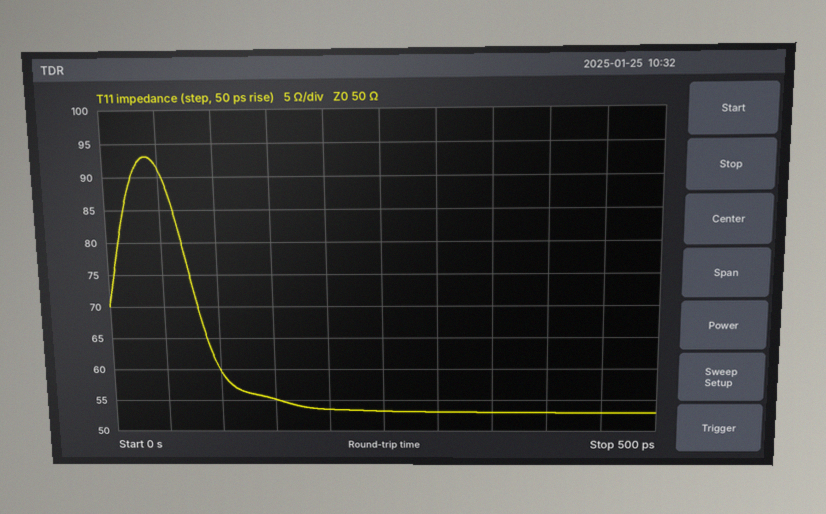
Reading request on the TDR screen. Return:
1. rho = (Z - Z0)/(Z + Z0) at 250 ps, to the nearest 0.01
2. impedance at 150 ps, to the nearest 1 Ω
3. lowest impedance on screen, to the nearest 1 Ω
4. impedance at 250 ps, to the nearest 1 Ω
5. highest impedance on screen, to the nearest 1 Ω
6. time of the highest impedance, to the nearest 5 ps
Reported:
+0.03
55 Ω
53 Ω
53 Ω
93 Ω
40 ps
